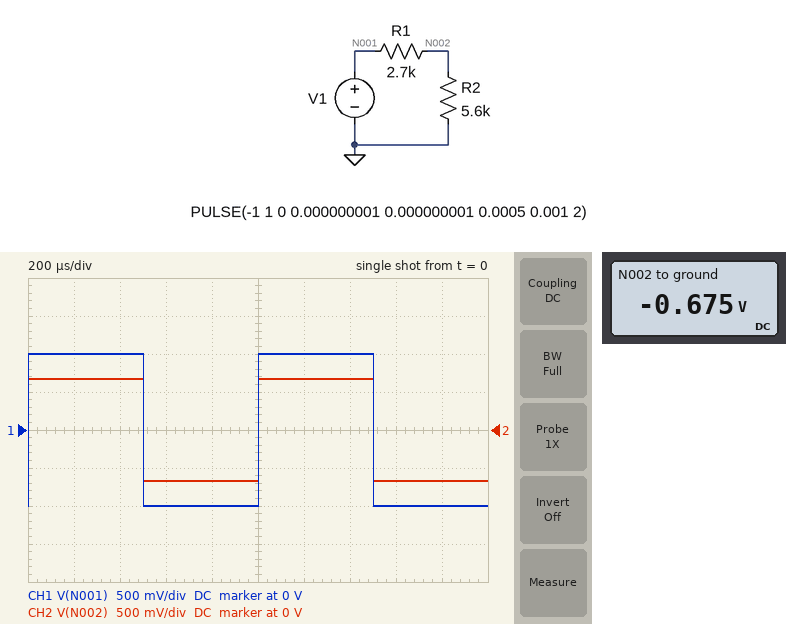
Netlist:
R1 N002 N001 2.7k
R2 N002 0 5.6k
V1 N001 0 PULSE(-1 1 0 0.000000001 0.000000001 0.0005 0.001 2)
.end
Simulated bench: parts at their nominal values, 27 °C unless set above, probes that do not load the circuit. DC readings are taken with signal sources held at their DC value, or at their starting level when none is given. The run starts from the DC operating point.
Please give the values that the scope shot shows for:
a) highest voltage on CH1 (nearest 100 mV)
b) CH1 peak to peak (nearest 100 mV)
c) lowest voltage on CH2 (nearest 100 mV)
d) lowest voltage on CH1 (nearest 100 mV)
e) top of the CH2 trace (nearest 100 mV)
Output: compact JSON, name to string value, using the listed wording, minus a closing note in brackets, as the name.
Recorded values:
{"highest voltage on CH1": "1.0 V", "CH1 peak to peak": "2.0 V", "lowest voltage on CH2": "-700 mV", "lowest voltage on CH1": "-1.0 V", "top of the CH2 trace": "700 mV"}
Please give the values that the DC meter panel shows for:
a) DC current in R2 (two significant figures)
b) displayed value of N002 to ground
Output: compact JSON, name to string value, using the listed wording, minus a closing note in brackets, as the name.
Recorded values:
{"DC current in R2": "120 µA", "displayed value of N002 to ground": "-0.675 V"}
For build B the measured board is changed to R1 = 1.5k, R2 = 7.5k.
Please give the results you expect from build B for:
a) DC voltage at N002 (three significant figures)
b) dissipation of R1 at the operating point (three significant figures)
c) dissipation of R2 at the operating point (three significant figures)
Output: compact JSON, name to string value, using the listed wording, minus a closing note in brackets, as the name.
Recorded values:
{"DC voltage at N002": "-833 mV", "dissipation of R1 at the operating point": "18.5 µW", "dissipation of R2 at the operating point": "92.6 µW"}
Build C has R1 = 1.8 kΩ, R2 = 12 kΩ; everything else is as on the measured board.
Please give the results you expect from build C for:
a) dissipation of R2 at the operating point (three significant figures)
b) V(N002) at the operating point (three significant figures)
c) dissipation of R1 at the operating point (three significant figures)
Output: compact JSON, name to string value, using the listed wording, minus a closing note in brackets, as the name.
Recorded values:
{"dissipation of R2 at the operating point": "63.0 µW", "V(N002) at the operating point": "-870 mV", "dissipation of R1 at the operating point": "9.45 µW"}
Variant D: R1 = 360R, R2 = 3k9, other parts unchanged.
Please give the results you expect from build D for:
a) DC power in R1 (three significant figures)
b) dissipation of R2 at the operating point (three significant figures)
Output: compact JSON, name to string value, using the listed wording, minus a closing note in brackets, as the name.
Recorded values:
{"DC power in R1": "19.8 µW", "dissipation of R2 at the operating point": "215 µW"}
